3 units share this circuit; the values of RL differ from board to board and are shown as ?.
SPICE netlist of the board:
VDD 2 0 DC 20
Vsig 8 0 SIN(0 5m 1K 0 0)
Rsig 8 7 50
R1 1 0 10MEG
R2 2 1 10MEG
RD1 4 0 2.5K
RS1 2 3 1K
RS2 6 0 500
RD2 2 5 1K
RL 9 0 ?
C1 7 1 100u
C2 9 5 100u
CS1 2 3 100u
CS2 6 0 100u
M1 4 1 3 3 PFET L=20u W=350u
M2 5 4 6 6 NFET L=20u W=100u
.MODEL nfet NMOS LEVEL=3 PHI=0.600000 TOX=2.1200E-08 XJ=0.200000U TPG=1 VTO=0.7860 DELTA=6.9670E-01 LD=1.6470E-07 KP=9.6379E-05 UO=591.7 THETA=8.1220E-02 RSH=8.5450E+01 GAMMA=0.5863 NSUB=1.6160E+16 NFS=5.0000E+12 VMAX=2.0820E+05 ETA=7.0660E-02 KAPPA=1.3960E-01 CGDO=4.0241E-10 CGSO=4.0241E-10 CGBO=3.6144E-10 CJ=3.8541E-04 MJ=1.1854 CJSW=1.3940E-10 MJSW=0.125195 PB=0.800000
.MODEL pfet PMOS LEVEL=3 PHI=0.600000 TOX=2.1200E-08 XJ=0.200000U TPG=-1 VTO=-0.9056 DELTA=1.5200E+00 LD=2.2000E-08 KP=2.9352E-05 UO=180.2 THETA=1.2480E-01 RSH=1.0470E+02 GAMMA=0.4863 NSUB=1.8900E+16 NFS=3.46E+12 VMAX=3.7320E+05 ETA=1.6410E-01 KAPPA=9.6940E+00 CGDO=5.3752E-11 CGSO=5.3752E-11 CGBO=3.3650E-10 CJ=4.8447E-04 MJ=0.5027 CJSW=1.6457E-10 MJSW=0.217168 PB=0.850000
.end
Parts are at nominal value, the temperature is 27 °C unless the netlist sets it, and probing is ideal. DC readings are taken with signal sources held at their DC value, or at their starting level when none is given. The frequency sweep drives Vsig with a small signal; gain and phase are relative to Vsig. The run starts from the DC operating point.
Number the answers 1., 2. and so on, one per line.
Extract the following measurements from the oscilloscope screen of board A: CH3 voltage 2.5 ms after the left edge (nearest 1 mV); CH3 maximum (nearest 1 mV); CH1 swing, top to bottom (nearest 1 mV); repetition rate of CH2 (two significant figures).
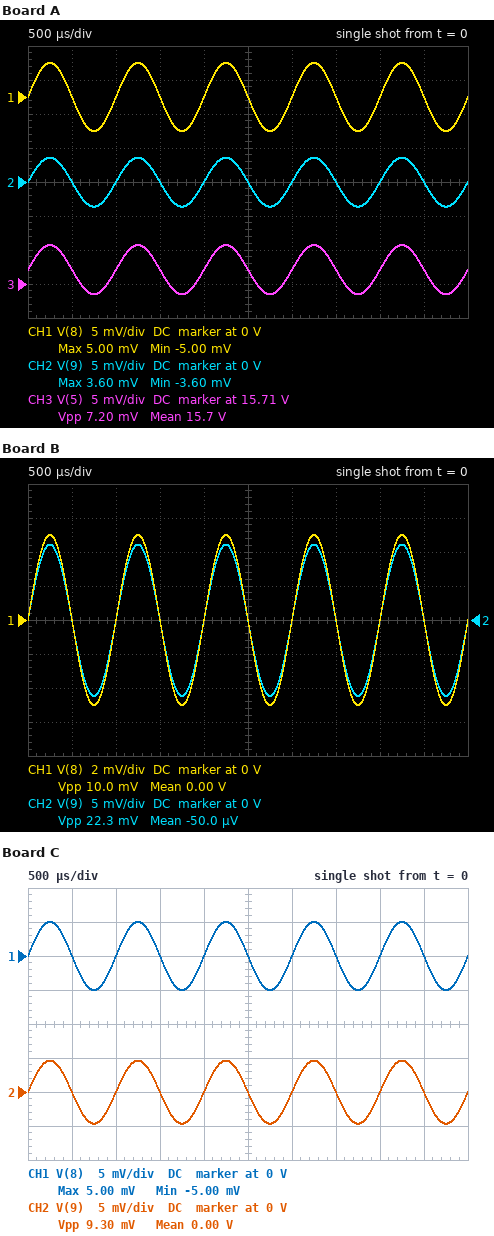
1. 15.717 V
2. 15.721 V
3. 10 mV
4. 1.0 kHz
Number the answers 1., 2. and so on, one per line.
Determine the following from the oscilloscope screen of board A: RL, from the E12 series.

1. 330 Ω
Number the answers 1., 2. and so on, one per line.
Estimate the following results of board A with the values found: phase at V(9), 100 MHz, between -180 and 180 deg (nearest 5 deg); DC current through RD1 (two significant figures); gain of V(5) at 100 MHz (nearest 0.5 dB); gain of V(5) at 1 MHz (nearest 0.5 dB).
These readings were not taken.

1. -110 deg
2. 3.6 mA
3. -15.0 dB
4. -3.0 dB
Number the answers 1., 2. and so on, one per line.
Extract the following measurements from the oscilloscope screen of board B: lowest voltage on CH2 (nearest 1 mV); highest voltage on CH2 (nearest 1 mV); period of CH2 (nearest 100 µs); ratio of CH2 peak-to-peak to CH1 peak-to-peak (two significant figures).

1. -11 mV
2. 11 mV
3. 1.0 ms
4. 2.2
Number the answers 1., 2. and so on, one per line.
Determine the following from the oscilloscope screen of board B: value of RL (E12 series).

1. 3.3 kΩ
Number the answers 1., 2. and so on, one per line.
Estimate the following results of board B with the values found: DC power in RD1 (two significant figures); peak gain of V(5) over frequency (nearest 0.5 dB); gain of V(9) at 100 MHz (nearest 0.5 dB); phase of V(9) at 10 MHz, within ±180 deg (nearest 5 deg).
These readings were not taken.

1. 32 mW
2. 7.0 dB
3. -5.5 dB
4. -25 deg
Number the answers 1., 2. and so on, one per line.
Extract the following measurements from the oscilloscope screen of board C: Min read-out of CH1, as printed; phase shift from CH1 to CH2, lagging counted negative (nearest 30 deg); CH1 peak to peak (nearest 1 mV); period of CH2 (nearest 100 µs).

1. -5.00 mV
2. 0 deg
3. 10 mV
4. 1.0 ms
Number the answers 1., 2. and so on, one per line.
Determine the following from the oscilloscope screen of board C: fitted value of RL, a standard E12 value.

1. 470 Ω
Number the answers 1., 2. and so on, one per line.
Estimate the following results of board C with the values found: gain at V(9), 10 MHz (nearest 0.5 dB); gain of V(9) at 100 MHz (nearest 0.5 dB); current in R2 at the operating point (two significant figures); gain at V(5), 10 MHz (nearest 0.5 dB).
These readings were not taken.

1. -1.0 dB
2. -13.0 dB
3. 1.0 µA
4. -1.0 dB
